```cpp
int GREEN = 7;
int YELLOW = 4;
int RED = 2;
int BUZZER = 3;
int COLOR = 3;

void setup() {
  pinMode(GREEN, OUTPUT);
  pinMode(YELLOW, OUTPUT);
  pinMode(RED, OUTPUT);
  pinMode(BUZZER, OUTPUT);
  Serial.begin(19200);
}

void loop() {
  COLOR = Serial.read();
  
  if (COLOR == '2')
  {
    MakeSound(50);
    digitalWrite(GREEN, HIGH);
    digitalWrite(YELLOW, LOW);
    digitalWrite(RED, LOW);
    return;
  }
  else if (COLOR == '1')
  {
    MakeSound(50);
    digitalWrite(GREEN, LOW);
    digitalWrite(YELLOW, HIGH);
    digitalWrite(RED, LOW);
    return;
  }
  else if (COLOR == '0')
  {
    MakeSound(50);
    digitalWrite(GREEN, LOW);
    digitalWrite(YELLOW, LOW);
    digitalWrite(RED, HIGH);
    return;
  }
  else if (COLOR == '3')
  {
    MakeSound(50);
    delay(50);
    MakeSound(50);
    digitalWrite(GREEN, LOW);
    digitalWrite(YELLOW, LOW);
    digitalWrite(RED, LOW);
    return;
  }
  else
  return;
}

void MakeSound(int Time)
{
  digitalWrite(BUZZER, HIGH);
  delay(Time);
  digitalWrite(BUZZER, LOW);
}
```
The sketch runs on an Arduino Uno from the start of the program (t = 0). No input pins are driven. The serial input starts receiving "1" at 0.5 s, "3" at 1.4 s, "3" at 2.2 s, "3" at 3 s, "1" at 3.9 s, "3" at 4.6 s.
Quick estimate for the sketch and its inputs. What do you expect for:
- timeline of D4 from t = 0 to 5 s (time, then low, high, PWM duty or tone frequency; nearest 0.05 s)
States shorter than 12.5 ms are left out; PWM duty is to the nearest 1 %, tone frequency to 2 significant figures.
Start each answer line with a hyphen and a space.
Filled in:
- 0 s low; 0.55 s high; 1.55 s low; 3.95 s high; 4.75 s low
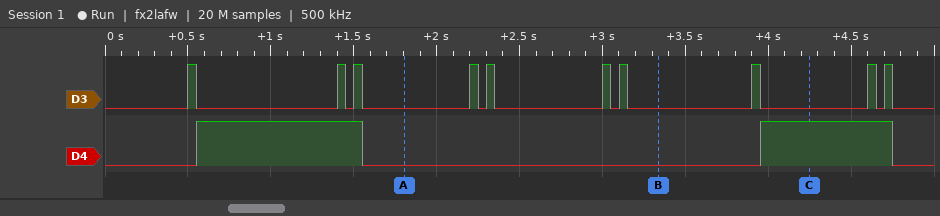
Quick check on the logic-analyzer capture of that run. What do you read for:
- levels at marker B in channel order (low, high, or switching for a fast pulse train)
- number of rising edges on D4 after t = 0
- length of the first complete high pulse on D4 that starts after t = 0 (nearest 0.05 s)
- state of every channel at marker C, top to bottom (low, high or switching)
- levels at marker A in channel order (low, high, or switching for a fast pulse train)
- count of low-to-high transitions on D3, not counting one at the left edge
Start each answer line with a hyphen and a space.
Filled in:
- D3 low, D4 low
- 2
- 1.00 s
- D3 low, D4 high
- D3 low, D4 low
- 10
